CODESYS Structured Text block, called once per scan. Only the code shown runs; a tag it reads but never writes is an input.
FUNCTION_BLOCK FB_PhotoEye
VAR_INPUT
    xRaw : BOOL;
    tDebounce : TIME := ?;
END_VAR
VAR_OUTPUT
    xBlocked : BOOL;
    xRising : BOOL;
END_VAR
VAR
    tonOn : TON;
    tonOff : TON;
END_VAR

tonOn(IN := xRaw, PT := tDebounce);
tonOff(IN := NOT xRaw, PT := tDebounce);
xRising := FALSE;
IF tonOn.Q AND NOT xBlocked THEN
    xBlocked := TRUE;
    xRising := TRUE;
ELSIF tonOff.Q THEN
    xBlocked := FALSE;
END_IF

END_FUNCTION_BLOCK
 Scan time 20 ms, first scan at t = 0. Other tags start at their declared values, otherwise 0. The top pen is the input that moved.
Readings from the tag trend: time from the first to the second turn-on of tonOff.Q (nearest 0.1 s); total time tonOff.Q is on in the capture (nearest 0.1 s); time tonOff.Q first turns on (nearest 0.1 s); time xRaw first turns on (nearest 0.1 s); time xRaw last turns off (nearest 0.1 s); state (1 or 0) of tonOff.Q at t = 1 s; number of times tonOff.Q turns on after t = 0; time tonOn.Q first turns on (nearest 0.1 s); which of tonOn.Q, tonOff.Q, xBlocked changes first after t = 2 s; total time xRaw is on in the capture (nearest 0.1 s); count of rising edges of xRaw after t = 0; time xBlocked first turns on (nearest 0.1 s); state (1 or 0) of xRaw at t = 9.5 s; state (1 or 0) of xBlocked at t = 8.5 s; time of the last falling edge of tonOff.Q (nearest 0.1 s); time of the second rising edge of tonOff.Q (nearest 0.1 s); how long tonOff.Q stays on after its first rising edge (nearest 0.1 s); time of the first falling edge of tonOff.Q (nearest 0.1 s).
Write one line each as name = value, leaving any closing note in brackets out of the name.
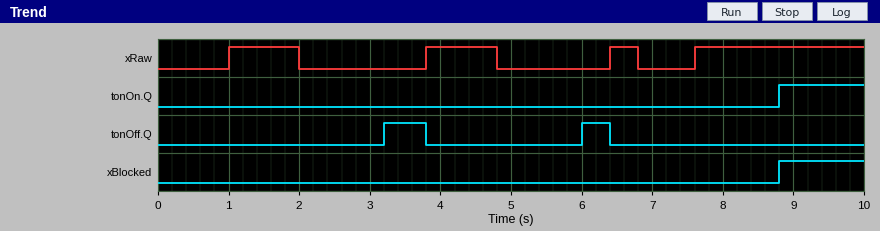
time from the first to the second turn-on of tonOff.Q = 2.8 s
total time tonOff.Q is on in the capture = 1.0 s
time tonOff.Q first turns on = 3.2 s
time xRaw first turns on = 1.0 s
time xRaw last turns off = 6.8 s
state (1 or 0) of tonOff.Q at t = 1 s = 0
number of times tonOff.Q turns on after t = 0 = 2
time tonOn.Q first turns on = 8.8 s
which of tonOn.Q, tonOff.Q, xBlocked changes first after t = 2 s = tonOff.Q
total time xRaw is on in the capture = 4.8 s
count of rising edges of xRaw after t = 0 = 4
time xBlocked first turns on = 8.8 s
state (1 or 0) of xRaw at t = 9.5 s = 1
state (1 or 0) of xBlocked at t = 8.5 s = 0
time of the last falling edge of tonOff.Q = 6.4 s
time of the second rising edge of tonOff.Q = 6.0 s
how long tonOff.Q stays on after its first rising edge = 0.6 s
time of the first falling edge of tonOff.Q = 3.8 s
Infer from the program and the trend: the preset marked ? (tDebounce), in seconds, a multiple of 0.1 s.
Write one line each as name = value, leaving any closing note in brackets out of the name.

the preset marked ? (tDebounce), in seconds, a multiple of 0.1 s = 1.2 s
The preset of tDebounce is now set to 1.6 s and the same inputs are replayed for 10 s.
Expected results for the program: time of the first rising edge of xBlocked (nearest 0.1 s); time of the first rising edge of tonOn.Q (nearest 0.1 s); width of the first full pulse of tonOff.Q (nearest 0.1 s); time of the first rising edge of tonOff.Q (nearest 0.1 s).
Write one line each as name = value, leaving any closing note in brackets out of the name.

time of the first rising edge of xBlocked = 9.2 s
time of the first rising edge of tonOn.Q = 9.2 s
width of the first full pulse of tonOff.Q = 0.2 s
time of the first rising edge of tonOff.Q = 3.6 s
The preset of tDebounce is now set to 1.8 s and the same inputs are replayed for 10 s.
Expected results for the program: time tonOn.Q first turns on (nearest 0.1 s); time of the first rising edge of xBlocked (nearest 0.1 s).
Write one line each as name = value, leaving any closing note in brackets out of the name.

time tonOn.Q first turns on = 9.4 s
time of the first rising edge of xBlocked = 9.4 s
